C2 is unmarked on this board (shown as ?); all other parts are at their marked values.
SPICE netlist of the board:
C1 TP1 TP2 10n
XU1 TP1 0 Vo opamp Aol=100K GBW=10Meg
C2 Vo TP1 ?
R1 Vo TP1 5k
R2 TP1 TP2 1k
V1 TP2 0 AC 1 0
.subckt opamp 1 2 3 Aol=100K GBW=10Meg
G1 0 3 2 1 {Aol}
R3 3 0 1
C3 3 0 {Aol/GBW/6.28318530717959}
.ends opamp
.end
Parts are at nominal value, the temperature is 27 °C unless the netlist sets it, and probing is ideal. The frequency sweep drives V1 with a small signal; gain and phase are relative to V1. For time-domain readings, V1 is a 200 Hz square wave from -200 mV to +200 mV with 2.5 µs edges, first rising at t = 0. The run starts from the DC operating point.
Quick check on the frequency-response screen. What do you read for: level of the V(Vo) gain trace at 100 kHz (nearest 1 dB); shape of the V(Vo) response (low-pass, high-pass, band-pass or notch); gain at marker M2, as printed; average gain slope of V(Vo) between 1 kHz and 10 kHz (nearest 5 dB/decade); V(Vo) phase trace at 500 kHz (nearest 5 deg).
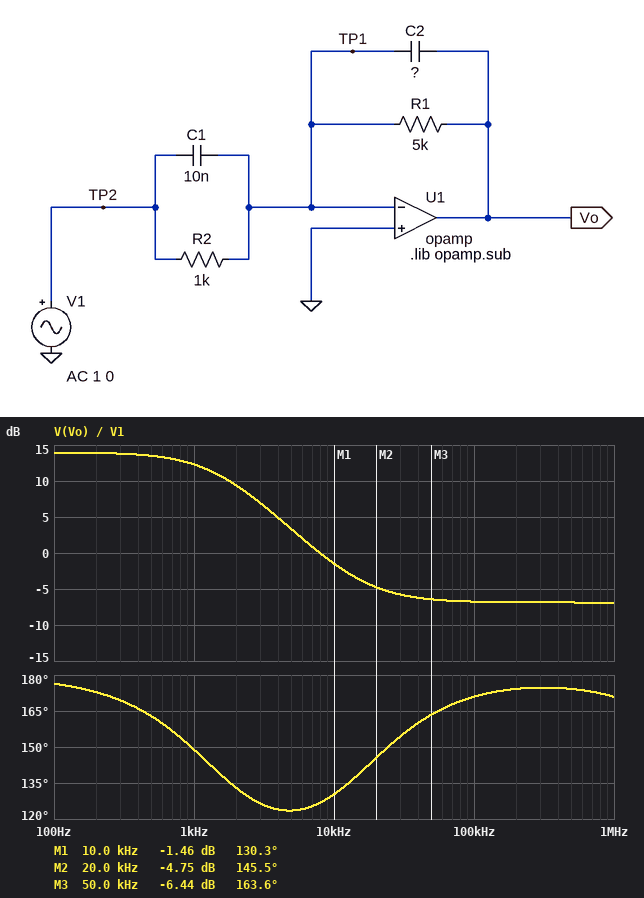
-7 dB
low-pass
-4.75 dB
-15 dB/decade
175 deg
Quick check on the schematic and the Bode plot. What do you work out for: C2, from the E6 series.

22 nF
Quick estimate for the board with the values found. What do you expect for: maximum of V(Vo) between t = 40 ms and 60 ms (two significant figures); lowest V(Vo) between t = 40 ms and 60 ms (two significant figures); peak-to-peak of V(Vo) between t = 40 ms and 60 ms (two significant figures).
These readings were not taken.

1.0 V
-1.0 V
2.0 V
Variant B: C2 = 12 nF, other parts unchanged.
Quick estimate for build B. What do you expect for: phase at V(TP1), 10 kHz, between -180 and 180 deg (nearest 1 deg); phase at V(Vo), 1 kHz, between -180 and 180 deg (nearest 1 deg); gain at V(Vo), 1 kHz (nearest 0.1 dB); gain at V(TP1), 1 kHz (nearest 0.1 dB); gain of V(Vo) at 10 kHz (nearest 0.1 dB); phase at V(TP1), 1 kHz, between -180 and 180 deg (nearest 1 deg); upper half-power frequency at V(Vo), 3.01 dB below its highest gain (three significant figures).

46 deg
163 deg
13.4 dB
-66.5 dB
3.6 dB
67 deg
2.73 kHz
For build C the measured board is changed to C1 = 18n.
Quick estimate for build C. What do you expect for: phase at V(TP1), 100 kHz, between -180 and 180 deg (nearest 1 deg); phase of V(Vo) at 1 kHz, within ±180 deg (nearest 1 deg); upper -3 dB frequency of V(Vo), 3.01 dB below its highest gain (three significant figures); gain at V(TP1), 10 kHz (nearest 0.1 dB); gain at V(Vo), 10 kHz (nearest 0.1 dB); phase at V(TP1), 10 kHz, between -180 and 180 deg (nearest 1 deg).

85 deg
152 deg
1.49 kHz
-59.3 dB
0.7 dB
56 deg
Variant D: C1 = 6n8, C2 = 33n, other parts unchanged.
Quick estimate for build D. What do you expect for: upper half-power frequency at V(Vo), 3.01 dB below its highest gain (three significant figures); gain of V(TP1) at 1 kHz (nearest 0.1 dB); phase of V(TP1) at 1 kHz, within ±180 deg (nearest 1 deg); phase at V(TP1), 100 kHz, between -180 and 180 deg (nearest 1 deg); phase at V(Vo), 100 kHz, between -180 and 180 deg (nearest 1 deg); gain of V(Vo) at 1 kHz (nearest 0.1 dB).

966 Hz
-69.1 dB
41 deg
77 deg
167 deg
10.8 dB
